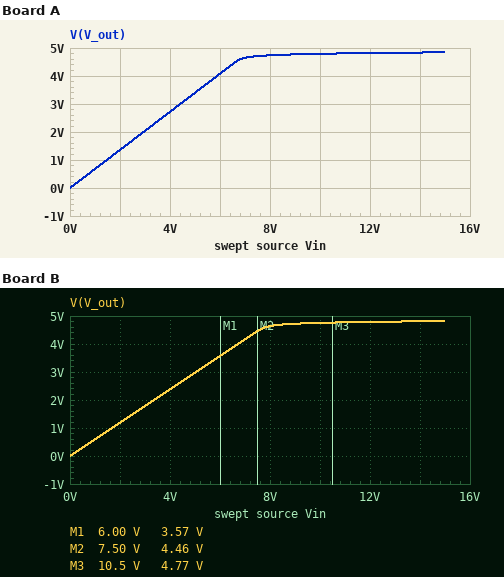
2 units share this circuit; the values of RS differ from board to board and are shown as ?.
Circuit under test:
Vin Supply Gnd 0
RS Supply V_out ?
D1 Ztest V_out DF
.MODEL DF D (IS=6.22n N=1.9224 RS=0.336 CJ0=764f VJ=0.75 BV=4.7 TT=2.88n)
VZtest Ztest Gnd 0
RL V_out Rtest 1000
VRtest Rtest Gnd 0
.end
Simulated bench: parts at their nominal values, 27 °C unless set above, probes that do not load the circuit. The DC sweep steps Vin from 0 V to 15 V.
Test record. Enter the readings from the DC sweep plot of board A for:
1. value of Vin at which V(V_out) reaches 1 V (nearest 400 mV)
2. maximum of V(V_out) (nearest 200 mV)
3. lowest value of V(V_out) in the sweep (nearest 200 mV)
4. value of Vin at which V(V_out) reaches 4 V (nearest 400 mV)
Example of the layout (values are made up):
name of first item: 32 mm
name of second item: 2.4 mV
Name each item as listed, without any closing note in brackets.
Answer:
value of Vin at which V(V_out) reaches 1 V: 1.6 V
maximum of V(V_out): 4.8 V
lowest value of V(V_out) in the sweep: 0 V
value of Vin at which V(V_out) reaches 4 V: 6.0 V
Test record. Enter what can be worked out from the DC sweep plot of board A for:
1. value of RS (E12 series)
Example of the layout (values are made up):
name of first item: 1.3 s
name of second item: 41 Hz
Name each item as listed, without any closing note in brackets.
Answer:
value of RS: 470 Ω
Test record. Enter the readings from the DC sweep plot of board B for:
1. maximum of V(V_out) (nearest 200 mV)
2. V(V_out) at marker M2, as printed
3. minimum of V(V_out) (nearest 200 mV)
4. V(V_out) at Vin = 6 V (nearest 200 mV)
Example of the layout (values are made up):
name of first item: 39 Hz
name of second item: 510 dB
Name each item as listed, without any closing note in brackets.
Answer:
maximum of V(V_out): 4.8 V
V(V_out) at marker M2, as printed: 4.46 V
minimum of V(V_out): 0 V
V(V_out) at Vin = 6 V: 3.6 V
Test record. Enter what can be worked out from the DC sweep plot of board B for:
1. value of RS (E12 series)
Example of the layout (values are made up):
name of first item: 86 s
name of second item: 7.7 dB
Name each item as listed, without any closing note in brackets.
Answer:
value of RS: 680 Ω
